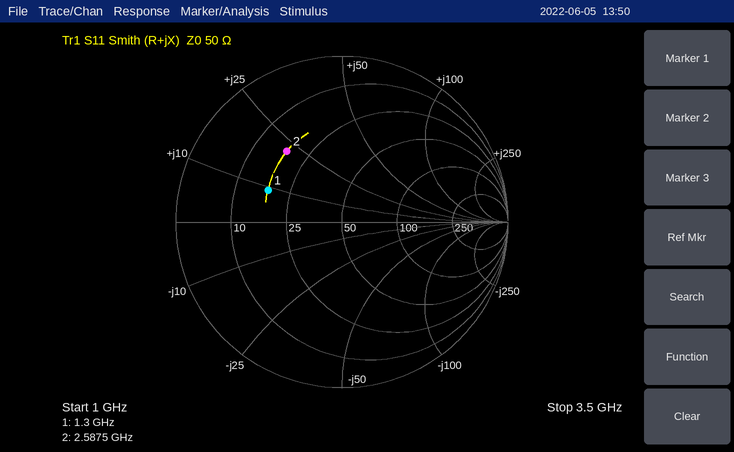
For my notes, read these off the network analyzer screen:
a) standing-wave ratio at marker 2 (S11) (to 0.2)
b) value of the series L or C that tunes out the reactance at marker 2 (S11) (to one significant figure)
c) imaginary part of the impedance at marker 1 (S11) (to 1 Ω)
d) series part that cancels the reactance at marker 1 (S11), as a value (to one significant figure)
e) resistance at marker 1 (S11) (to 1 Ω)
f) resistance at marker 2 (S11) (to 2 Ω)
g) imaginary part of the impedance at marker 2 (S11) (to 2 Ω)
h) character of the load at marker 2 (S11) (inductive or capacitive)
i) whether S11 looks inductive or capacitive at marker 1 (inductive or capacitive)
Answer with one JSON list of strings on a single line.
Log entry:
["3.4", "3 pF", "+9 Ω", "10 pF", "18 Ω", "18 Ω", "+22 Ω", "inductive", "inductive"]
